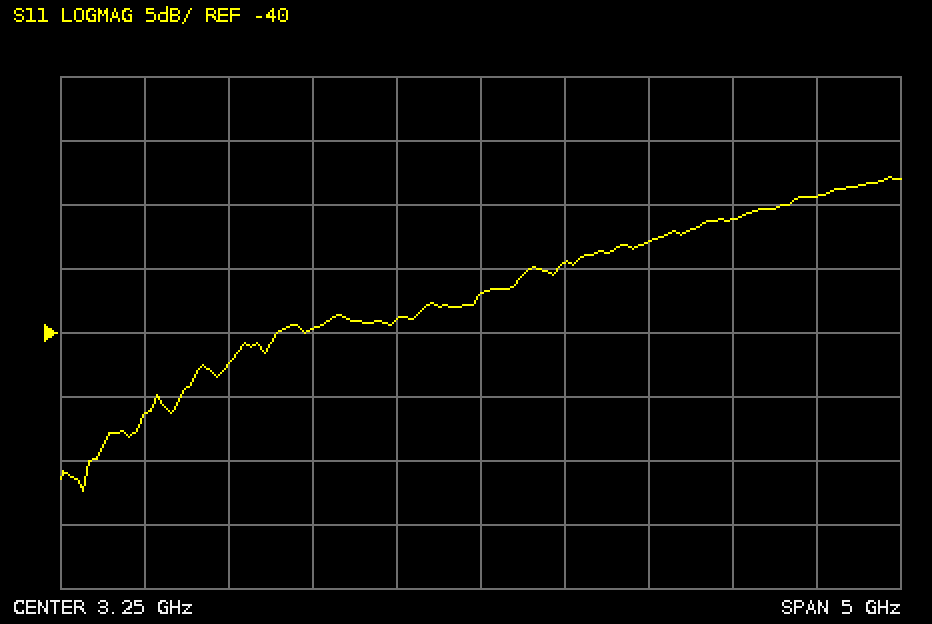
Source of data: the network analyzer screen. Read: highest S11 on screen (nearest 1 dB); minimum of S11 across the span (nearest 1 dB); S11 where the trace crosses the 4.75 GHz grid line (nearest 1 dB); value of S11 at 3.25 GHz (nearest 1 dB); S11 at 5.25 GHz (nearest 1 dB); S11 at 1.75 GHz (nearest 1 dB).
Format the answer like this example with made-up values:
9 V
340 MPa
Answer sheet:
-28 dB
-52 dB
-31 dB
-37 dB
-29 dB
-42 dB
